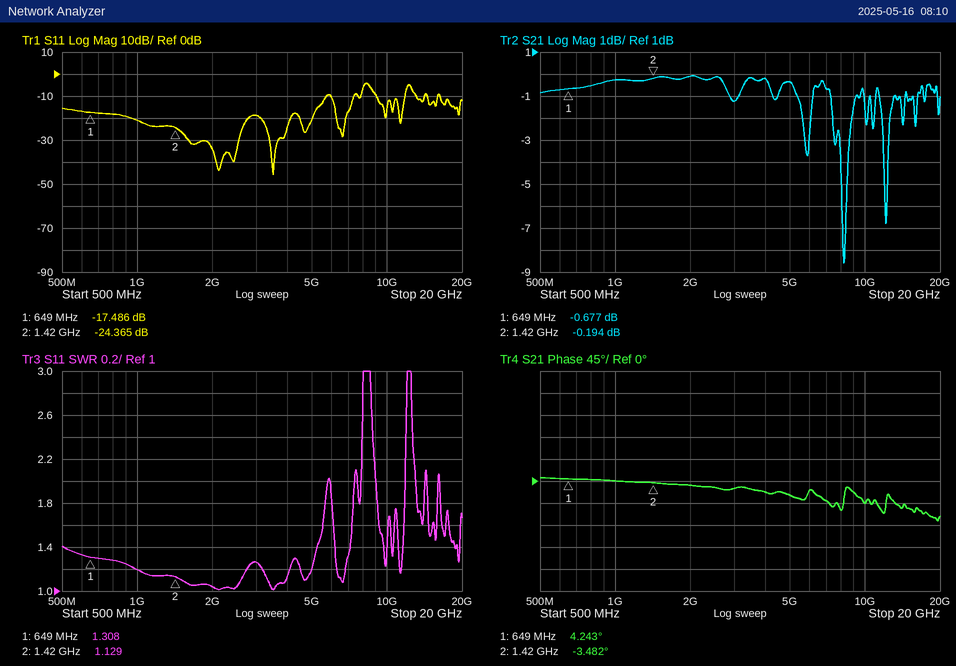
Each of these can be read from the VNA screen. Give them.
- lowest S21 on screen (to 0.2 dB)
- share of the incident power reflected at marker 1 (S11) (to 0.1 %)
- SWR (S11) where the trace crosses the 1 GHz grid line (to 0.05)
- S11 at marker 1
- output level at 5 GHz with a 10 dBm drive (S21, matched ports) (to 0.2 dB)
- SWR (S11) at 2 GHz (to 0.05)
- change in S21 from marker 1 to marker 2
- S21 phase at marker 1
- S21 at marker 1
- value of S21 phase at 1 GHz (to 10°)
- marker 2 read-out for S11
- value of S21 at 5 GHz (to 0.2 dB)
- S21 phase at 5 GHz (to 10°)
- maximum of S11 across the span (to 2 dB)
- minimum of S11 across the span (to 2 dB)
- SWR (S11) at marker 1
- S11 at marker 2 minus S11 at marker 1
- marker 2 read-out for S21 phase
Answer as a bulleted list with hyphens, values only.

- -8.6 dB
- 1.8 %
- 1.20
- -17.486 dB
- 9.6 dBm
- 1.05
- 0.483 dB
- 4.243°
- -0.677 dB
- 0°
- -24.365 dB
- -0.4 dB
- -30°
- -4 dB
- -46 dB
- 1.308
- -6.879 dB
- -3.482°
